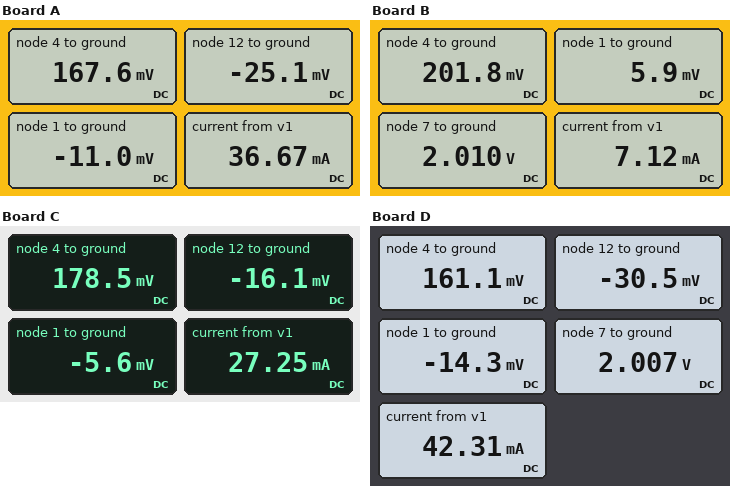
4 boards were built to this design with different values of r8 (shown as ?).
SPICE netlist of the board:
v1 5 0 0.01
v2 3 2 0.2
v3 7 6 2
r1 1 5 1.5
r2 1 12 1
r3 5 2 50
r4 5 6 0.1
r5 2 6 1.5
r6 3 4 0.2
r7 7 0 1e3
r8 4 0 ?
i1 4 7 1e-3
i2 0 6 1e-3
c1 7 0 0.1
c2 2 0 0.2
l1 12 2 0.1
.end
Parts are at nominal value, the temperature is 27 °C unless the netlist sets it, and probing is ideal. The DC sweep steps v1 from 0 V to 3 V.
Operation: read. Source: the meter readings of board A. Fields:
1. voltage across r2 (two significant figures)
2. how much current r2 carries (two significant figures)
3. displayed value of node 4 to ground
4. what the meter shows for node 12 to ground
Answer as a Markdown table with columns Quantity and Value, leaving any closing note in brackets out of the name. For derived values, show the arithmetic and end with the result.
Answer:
| Quantity | Value |
|---|---|
| voltage across r2 | -11 mV - (-25.1 mV) = 14 mV |
| how much current r2 carries | (-11 mV - (-25.1 mV)) / 1 Ω = 14 mA |
| displayed value of node 4 to ground | 167.6 mV |
| what the meter shows for node 12 to ground | -25.1 mV |
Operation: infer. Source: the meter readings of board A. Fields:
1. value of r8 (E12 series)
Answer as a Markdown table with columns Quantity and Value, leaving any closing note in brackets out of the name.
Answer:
| Quantity | Value |
|---|---|
| value of r8 | 4.7 Ω |
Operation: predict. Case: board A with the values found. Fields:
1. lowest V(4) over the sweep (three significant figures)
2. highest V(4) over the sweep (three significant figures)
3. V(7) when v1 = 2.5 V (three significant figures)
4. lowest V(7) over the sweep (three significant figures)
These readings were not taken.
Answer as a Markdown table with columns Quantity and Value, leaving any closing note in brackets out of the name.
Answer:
| Quantity | Value |
|---|---|
| lowest V(4) over the sweep | 160 mV |
| highest V(4) over the sweep | 2.57 V |
| V(7) when v1 = 2.5 V | 4.47 V |
| lowest V(7) over the sweep | 2.00 V |
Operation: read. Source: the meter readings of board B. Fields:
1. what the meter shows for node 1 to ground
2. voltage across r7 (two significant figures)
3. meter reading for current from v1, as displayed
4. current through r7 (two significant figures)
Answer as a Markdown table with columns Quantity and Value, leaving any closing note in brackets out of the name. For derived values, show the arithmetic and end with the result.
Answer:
| Quantity | Value |
|---|---|
| what the meter shows for node 1 to ground | 5.9 mV |
| voltage across r7 | 2.01 V = 2.0 V |
| meter reading for current from v1, as displayed | 7.12 mA |
| current through r7 | (2.01 V) / 1 kΩ = 2.0 mA |
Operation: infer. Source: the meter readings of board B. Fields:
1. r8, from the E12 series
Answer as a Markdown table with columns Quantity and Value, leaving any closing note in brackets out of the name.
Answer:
| Quantity | Value |
|---|---|
| r8, from the E12 series | 33 Ω |
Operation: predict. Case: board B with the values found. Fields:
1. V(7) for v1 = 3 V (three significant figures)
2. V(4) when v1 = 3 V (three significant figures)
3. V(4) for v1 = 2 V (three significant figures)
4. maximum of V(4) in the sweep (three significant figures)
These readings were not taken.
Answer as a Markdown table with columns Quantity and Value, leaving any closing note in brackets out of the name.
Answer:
| Quantity | Value |
|---|---|
| V(7) for v1 = 3 V | 4.99 V |
| V(4) when v1 = 3 V | 3.09 V |
| V(4) for v1 = 2 V | 2.12 V |
| maximum of V(4) in the sweep | 3.09 V |
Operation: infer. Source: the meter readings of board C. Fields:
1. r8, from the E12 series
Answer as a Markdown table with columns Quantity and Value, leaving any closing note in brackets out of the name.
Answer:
| Quantity | Value |
|---|---|
| r8, from the E12 series | 6.8 Ω |
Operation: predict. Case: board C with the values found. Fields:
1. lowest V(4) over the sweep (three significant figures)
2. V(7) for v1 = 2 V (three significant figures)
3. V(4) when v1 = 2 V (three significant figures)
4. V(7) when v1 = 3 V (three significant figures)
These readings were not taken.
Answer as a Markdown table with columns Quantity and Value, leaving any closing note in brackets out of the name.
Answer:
| Quantity | Value |
|---|---|
| lowest V(4) over the sweep | 170 mV |
| V(7) for v1 = 2 V | 3.98 V |
| V(4) when v1 = 2 V | 1.88 V |
| V(7) when v1 = 3 V | 4.98 V |
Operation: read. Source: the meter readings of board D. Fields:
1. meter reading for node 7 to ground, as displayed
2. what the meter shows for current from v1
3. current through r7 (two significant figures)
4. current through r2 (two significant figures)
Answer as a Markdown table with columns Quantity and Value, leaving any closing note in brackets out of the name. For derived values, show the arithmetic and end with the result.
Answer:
| Quantity | Value |
|---|---|
| meter reading for node 7 to ground, as displayed | 2.007 V |
| what the meter shows for current from v1 | 42.31 mA |
| current through r7 | (2.007 V) / 1 kΩ = 2.0 mA |
| current through r2 | (-14.3 mV - (-30.5 mV)) / 1 Ω = 16 mA |
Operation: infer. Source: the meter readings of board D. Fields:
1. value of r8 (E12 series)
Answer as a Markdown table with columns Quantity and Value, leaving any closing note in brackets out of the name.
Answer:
| Quantity | Value |
|---|---|
| value of r8 | 3.9 Ω |
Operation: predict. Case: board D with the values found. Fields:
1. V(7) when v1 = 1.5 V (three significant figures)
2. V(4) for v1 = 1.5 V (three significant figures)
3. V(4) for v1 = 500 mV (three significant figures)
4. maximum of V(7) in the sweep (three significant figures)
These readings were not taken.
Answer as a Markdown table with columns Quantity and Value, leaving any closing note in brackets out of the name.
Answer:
| Quantity | Value |
|---|---|
| V(7) when v1 = 1.5 V | 3.48 V |
| V(4) for v1 = 1.5 V | 1.31 V |
| V(4) for v1 = 500 mV | 539 mV |
| maximum of V(7) in the sweep | 4.96 V |
